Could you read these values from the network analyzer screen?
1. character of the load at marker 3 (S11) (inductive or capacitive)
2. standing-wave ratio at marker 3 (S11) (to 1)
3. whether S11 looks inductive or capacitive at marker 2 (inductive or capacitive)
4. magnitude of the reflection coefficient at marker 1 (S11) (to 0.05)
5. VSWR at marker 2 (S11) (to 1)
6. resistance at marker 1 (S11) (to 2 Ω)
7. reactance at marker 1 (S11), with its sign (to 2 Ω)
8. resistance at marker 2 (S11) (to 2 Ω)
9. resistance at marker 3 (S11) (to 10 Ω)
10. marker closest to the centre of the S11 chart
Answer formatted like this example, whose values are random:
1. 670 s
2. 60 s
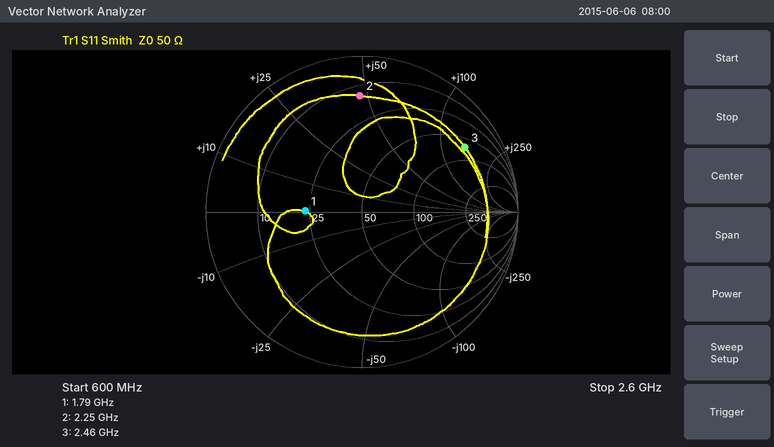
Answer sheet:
1. inductive
2. 8
3. inductive
4. 0.35
5. 7
6. 24 Ω
7. 0 Ω
8. 14 Ω
9. 70 Ω
10. marker 1
